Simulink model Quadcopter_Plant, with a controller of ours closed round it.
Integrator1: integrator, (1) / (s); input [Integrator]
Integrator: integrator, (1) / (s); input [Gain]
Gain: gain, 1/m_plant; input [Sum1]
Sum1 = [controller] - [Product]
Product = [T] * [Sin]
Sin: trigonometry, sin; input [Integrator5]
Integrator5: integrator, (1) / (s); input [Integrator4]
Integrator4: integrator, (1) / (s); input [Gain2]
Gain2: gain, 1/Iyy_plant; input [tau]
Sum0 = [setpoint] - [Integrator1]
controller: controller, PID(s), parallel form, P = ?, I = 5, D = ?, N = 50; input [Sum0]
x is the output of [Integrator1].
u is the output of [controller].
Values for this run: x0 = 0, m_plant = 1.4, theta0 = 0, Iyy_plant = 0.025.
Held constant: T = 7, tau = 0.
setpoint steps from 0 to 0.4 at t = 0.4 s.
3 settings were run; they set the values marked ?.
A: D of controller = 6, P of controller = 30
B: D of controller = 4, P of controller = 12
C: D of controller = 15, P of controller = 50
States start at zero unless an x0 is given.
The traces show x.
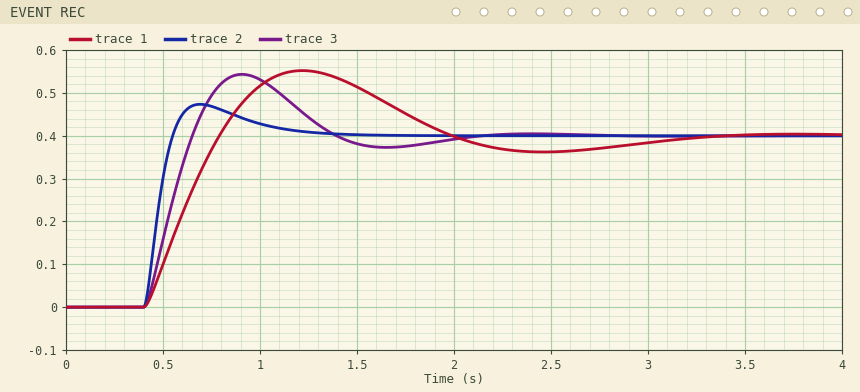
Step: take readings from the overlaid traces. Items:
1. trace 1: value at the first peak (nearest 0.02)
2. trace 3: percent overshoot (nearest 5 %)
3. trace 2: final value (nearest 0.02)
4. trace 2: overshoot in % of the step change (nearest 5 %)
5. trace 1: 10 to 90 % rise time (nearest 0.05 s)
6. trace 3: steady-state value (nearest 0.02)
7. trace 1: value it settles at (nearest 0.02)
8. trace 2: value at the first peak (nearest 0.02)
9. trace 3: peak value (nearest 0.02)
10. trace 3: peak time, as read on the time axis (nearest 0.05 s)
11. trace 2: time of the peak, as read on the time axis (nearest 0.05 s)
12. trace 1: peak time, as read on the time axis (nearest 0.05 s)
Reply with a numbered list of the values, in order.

1. 0.56
2. 35 %
3. 0.40
4. 20 %
5. 0.30 s
6. 0.40
7. 0.40
8. 0.48
9. 0.54
10. 0.90 s
11. 0.70 s
12. 1.20 s
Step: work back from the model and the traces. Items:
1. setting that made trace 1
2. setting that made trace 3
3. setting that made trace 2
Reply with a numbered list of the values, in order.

1. B
2. A
3. C
